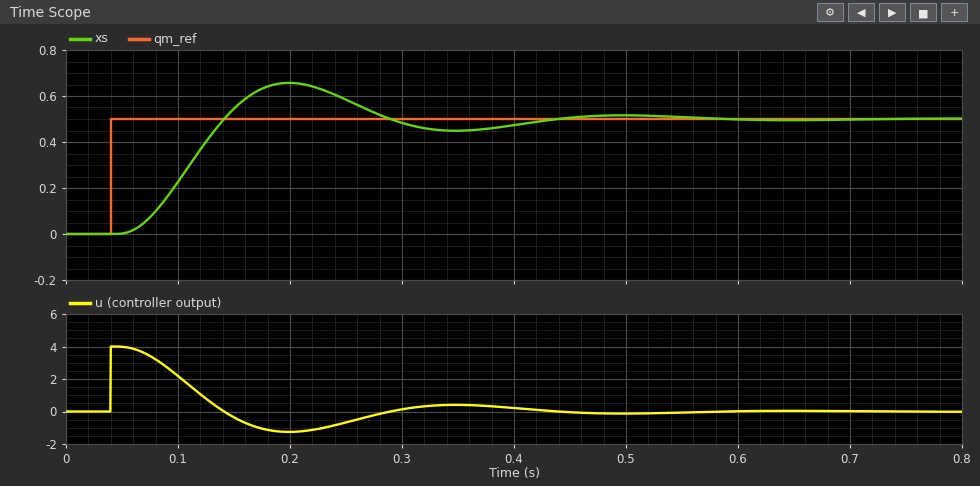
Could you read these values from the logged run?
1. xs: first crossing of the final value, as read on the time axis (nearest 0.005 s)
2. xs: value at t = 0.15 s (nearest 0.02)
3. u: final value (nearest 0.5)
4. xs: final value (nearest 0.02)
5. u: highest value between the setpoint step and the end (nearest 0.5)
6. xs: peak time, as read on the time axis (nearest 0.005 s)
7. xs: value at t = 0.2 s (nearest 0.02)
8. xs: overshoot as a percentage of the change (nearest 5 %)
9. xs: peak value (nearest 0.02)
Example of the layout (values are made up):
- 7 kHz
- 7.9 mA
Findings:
- 0.140 s
- 0.54
- 0.0
- 0.50
- 4.0
- 0.200 s
- 0.66
- 30 %
- 0.66
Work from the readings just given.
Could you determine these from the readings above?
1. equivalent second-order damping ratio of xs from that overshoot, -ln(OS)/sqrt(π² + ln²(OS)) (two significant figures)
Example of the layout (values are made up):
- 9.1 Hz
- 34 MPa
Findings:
- 0.36
